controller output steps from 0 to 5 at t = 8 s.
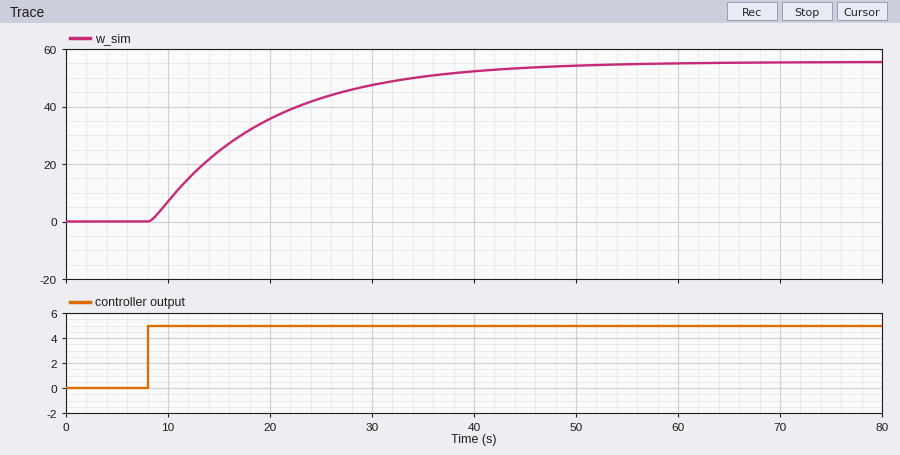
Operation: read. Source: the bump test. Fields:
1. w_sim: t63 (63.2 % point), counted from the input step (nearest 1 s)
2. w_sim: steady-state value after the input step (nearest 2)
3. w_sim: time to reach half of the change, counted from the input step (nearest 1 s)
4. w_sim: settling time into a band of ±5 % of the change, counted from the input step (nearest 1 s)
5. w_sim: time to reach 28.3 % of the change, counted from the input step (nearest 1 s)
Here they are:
12 s
56
8 s
34 s
4 s
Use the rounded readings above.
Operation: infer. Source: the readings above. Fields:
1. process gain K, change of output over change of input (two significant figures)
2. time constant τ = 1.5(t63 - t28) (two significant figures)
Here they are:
11
12 s
